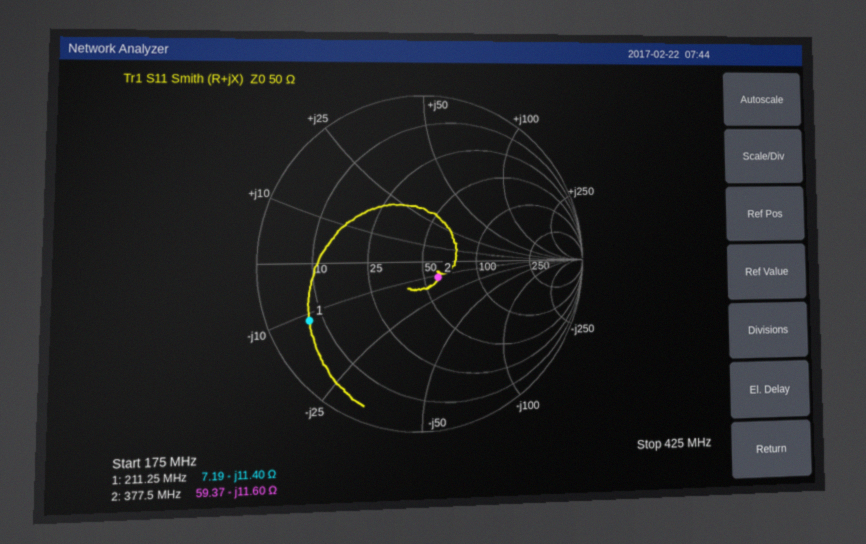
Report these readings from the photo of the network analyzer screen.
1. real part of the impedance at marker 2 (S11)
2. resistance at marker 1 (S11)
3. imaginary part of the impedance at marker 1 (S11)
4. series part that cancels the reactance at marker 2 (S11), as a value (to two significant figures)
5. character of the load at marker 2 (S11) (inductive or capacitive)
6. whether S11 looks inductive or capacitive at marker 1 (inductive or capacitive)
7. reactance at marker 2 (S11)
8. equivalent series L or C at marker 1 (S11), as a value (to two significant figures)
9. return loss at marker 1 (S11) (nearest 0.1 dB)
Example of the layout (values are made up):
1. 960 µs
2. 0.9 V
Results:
1. 59.37 Ω
2. 7.19 Ω
3. -11.40 Ω
4. 4.9 nH
5. capacitive
6. capacitive
7. -11.60 Ω
8. 66 pF
9. 2.4 dB
